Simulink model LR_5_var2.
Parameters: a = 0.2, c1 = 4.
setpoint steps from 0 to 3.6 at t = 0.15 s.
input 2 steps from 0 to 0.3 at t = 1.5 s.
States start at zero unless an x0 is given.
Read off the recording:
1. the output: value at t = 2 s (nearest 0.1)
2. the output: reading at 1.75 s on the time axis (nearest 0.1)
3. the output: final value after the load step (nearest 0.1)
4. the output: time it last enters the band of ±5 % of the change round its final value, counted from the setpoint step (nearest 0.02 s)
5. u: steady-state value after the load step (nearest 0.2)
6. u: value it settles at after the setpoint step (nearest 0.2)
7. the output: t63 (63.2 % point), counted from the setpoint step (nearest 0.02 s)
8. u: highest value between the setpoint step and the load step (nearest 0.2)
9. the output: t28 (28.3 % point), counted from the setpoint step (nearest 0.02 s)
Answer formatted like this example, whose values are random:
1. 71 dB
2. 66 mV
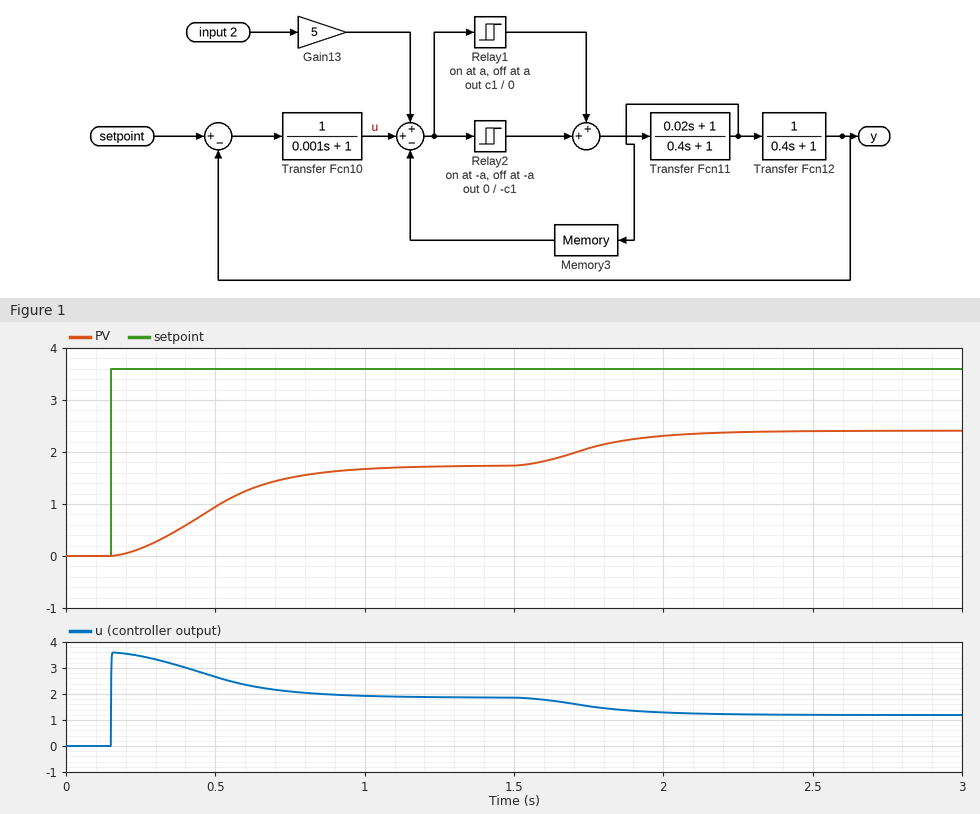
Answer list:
1. 2.3
2. 2.1
3. 2.4
4. 0.80 s
5. 1.2
6. 1.8
7. 0.40 s
8. 3.6
9. 0.22 s
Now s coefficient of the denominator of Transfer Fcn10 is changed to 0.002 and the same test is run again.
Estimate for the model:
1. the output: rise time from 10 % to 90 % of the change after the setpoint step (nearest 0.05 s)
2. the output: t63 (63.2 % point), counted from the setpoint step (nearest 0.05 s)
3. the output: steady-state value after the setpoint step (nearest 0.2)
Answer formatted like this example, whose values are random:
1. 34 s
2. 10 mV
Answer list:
1. 0.55 s
2. 0.40 s
3. 1.8
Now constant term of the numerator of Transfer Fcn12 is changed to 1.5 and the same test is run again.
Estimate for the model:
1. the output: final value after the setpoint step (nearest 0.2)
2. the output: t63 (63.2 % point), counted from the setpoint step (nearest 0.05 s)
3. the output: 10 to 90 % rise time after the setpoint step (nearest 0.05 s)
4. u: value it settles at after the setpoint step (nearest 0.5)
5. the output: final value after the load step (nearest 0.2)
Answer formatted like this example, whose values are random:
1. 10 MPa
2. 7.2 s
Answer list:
1. 2.0
2. 0.35 s
3. 0.45 s
4. 1.5
5. 3.0
